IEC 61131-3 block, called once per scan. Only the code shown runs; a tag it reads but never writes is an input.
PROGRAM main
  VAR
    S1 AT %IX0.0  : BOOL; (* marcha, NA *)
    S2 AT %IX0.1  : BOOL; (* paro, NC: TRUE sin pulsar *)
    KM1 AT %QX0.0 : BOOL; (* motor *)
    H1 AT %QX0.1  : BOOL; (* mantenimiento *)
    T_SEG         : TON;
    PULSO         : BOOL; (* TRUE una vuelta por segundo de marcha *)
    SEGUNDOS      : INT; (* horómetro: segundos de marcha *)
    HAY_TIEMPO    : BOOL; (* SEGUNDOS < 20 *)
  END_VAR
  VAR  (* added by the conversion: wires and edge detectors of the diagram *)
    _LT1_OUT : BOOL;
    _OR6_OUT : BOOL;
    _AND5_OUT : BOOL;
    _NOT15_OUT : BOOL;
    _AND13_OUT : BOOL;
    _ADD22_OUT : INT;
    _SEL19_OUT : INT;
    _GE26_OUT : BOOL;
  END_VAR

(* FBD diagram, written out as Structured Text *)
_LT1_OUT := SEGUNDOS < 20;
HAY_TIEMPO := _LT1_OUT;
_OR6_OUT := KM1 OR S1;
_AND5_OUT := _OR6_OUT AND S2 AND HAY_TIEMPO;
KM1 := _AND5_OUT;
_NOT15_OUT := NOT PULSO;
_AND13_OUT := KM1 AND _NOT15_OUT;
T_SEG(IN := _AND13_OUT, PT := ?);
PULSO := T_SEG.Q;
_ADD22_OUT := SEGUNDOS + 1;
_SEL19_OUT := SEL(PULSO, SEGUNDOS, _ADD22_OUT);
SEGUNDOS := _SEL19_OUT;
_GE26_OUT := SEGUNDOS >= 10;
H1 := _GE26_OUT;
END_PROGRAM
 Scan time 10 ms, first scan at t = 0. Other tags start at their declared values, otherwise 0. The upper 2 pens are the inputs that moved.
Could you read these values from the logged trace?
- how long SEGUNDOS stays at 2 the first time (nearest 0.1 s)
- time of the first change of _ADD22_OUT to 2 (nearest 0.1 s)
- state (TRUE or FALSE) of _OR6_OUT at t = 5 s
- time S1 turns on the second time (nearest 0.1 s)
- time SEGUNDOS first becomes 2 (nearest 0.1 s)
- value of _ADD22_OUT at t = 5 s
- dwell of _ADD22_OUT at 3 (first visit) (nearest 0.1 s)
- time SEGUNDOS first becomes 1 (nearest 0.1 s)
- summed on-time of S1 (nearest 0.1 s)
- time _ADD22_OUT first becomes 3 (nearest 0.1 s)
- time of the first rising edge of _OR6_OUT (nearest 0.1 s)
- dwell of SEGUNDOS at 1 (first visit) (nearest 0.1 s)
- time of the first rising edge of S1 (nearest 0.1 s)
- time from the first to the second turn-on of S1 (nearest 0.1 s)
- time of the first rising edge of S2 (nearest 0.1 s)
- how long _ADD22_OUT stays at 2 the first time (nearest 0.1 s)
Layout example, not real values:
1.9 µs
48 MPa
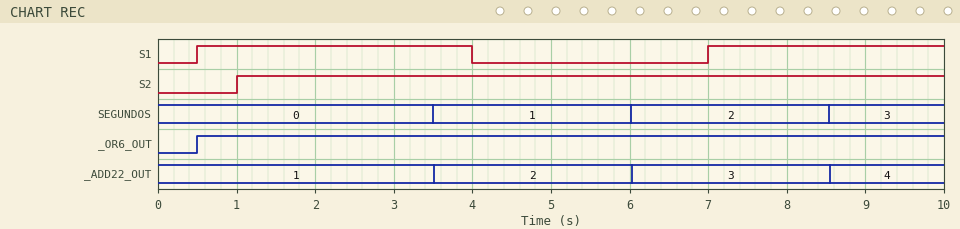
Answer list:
2.5 s
3.5 s
TRUE
7.0 s
6.0 s
2
2.5 s
3.5 s
6.5 s
6.0 s
0.5 s
2.5 s
0.5 s
6.5 s
1.0 s
2.5 s
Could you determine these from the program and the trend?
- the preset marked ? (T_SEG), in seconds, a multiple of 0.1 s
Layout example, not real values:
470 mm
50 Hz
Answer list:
2.5 s
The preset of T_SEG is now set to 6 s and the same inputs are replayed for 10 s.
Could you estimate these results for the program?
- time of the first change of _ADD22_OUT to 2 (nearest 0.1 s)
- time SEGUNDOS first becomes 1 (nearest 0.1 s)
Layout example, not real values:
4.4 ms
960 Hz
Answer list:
7.0 s
7.0 s
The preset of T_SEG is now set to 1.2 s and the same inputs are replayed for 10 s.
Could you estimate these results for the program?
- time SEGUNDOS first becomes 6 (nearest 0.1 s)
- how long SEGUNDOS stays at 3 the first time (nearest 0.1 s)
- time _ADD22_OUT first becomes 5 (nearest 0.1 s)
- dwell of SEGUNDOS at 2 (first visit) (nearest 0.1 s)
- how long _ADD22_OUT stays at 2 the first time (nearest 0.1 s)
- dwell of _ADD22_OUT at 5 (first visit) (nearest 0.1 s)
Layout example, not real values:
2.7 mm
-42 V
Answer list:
8.3 s
1.2 s
5.9 s
1.2 s
1.2 s
1.2 s
